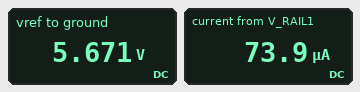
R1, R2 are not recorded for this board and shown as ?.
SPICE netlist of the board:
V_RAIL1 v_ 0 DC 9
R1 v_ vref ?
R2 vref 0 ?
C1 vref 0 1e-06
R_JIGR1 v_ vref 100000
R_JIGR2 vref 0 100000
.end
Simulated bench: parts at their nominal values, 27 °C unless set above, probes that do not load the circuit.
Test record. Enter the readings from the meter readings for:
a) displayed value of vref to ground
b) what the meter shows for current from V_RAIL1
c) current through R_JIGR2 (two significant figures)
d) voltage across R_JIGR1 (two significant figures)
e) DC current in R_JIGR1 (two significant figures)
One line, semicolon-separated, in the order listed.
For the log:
5.671 V; 73.9 µA; 57 µA; 3.3 V; 33 µA
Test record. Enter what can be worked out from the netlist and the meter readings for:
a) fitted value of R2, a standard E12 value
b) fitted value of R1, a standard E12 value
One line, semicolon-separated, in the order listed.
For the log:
330 kΩ; 82 kΩ
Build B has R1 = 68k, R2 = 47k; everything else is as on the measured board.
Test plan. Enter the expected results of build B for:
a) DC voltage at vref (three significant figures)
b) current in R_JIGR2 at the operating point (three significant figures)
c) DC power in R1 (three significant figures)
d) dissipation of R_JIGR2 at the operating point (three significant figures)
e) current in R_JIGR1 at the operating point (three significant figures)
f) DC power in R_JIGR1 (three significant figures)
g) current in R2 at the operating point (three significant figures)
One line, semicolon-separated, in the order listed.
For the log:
3.97 V; 39.7 µA; 372 µW; 158 µW; 50.3 µA; 253 µW; 84.5 µA
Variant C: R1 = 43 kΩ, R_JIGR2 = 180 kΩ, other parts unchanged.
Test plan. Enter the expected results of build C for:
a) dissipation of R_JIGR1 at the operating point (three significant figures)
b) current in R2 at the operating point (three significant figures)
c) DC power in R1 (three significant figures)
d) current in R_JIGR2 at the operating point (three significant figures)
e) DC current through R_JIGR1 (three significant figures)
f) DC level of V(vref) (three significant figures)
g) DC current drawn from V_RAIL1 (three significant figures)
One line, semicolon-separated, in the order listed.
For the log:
34.1 µW; 21.7 µA; 79.3 µW; 39.7 µA; 18.5 µA; 7.15 V; 61.4 µA
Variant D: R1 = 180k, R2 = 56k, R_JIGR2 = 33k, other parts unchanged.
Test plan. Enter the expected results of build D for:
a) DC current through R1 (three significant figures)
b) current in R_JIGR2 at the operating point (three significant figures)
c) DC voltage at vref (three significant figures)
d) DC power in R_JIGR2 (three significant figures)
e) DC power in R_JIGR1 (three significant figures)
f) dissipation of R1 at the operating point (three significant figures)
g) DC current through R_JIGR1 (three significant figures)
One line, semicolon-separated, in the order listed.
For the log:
37.8 µA; 66.6 µA; 2.20 V; 146 µW; 463 µW; 257 µW; 68.0 µA
